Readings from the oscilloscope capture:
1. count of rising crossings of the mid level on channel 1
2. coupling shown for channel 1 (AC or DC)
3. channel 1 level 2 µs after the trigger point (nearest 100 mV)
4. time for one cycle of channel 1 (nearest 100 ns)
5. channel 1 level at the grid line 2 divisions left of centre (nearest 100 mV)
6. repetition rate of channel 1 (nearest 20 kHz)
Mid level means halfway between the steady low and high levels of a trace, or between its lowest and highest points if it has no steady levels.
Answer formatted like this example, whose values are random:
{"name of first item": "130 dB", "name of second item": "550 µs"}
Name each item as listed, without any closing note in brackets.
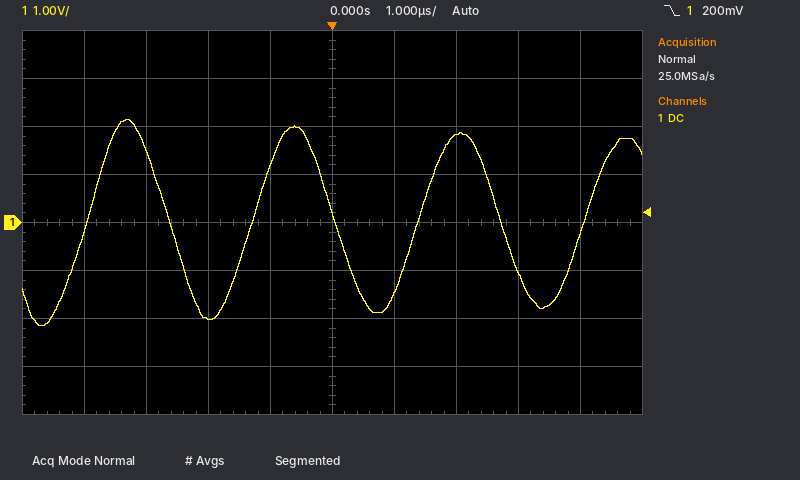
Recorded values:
{"count of rising crossings of the mid level on channel 1": "4", "coupling shown for channel 1": "DC", "channel 1 level 2 µs after the trigger point": "1.8 V", "time for one cycle of channel 1": "2.7 µs", "channel 1 level at the grid line 2 divisions left of centre": "-2.0 V", "repetition rate of channel 1": "380 kHz"}
